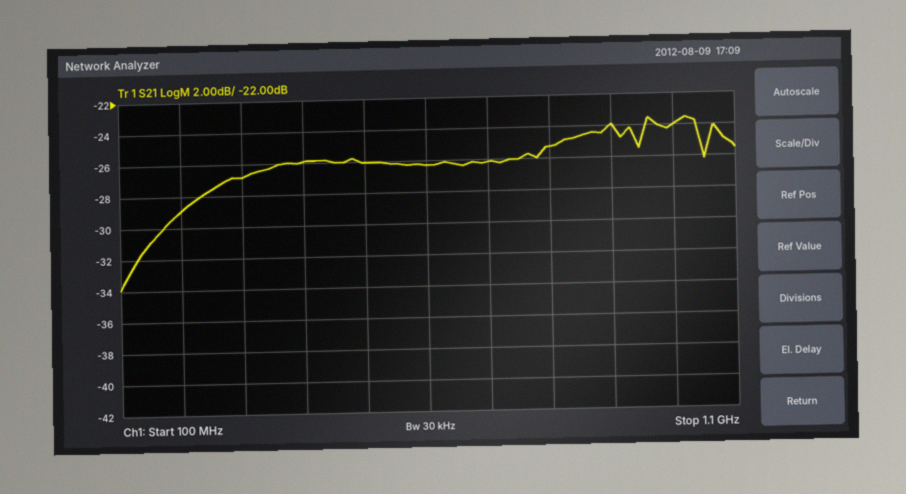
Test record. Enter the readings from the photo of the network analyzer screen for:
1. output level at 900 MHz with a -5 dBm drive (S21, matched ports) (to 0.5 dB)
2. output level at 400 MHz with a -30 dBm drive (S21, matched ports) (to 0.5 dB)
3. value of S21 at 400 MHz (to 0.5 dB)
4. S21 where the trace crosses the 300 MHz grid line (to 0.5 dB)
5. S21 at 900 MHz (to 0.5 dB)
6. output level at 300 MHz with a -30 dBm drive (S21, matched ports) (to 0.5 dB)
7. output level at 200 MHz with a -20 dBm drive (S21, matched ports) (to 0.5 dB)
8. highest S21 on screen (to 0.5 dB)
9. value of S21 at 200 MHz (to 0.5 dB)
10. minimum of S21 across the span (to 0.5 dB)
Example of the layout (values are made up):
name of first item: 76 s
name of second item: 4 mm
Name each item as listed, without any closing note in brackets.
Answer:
output level at 900 MHz with a -5 dBm drive (S21, matched ports): -29.0 dBm
output level at 400 MHz with a -30 dBm drive (S21, matched ports): -56.0 dBm
value of S21 at 400 MHz: -26.0 dB
S21 where the trace crosses the 300 MHz grid line: -27.0 dB
S21 at 900 MHz: -24.0 dB
output level at 300 MHz with a -30 dBm drive (S21, matched ports): -57.0 dBm
output level at 200 MHz with a -20 dBm drive (S21, matched ports): -49.0 dBm
highest S21 on screen: -23.5 dB
value of S21 at 200 MHz: -29.0 dB
minimum of S21 across the span: -34.0 dB
